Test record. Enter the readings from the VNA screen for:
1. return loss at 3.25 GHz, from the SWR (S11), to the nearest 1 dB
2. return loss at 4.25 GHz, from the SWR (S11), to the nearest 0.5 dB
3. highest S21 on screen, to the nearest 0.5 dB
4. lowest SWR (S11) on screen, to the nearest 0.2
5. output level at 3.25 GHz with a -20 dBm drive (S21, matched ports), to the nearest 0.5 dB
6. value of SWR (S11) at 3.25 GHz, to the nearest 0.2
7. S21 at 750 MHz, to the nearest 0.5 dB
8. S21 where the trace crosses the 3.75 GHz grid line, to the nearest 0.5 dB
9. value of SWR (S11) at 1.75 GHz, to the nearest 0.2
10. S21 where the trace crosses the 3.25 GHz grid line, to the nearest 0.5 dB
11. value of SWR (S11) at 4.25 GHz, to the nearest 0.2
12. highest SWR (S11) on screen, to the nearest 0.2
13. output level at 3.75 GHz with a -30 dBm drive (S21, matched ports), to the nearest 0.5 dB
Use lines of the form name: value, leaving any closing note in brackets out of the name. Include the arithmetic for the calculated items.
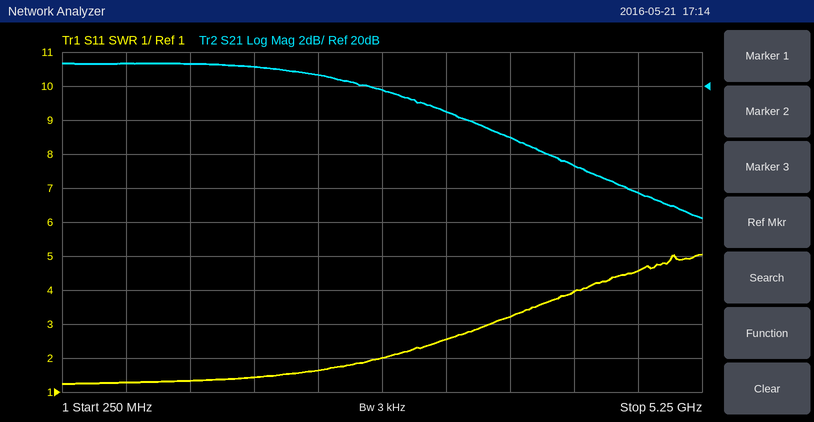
return loss at 3.25 GHz, from the SWR (S11), to the nearest 1 dB: −20 log10((2.6 − 1)/(2.6 + 1)) ≈ 7 dB
return loss at 4.25 GHz, from the SWR (S11), to the nearest 0.5 dB: −20 log10((4 − 1)/(4 + 1)) ≈ 4.44 dB, so 4.5 dB to the nearest 0.5 dB
highest S21 on screen, to the nearest 0.5 dB: 21.5 dB
lowest SWR (S11) on screen, to the nearest 0.2: 1.2
output level at 3.25 GHz with a -20 dBm drive (S21, matched ports), to the nearest 0.5 dB: -20 dBm + (18.5 dB) = -1.5 dBm
value of SWR (S11) at 3.25 GHz, to the nearest 0.2: 2.6
S21 at 750 MHz, to the nearest 0.5 dB: 21.5 dB
S21 where the trace crosses the 3.75 GHz grid line, to the nearest 0.5 dB: 17.0 dB
value of SWR (S11) at 1.75 GHz, to the nearest 0.2: 1.4
S21 where the trace crosses the 3.25 GHz grid line, to the nearest 0.5 dB: 18.5 dB
value of SWR (S11) at 4.25 GHz, to the nearest 0.2: 4.0
highest SWR (S11) on screen, to the nearest 0.2: 5.0
output level at 3.75 GHz with a -30 dBm drive (S21, matched ports), to the nearest 0.5 dB: -30 dBm + (17.0 dB) = -13.0 dBm
